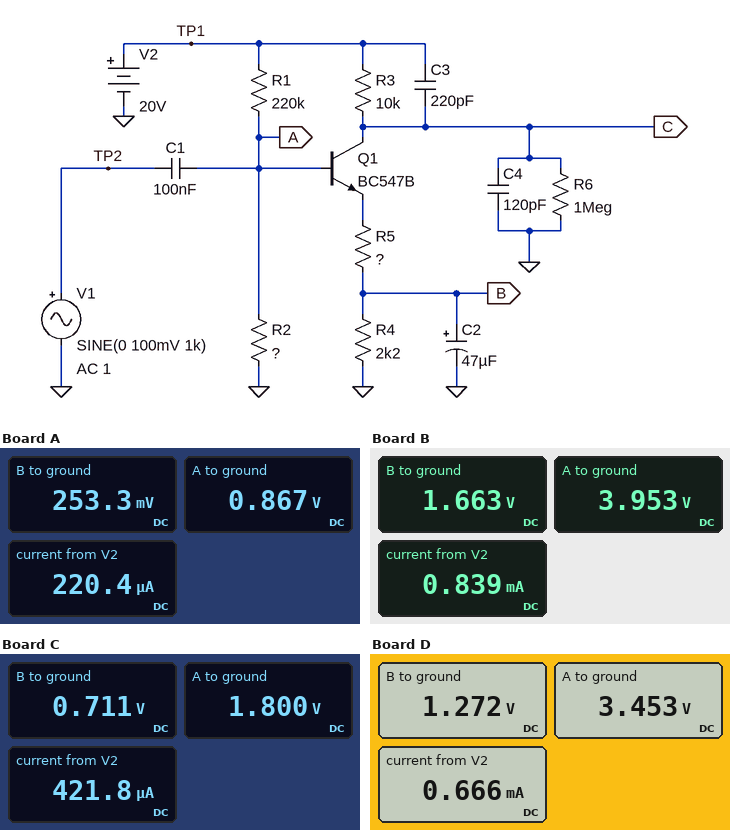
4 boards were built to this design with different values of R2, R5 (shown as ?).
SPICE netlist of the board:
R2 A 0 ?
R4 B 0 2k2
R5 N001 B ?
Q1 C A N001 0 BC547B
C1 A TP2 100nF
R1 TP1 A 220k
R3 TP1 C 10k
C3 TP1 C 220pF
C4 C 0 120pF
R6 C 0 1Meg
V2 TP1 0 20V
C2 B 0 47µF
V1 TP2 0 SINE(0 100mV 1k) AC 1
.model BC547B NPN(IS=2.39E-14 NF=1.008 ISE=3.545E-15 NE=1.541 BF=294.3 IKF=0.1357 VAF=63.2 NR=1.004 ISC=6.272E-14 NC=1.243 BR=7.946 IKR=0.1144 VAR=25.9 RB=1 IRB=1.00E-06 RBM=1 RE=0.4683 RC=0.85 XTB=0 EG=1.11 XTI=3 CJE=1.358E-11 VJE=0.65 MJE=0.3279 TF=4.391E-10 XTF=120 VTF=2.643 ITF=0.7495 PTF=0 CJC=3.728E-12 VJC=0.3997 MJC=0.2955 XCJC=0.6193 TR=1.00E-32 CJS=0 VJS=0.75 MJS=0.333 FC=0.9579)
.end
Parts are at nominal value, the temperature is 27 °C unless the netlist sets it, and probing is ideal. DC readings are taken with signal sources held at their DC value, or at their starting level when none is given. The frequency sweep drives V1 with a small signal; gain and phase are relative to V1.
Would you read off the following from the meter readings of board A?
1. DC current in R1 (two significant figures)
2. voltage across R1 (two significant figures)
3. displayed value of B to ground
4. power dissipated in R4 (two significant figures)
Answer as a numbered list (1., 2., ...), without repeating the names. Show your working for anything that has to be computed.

1. (20 V - 867 mV) / 220 kΩ = 87 µA
2. 20 V - 867 mV = 19 V
3. 253.3 mV
4. (253.3 mV)^2 / 2.2 kΩ = 29 µW
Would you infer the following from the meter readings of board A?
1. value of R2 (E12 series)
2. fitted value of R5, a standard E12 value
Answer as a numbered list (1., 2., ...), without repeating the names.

1. 10 kΩ
2. 330 Ω
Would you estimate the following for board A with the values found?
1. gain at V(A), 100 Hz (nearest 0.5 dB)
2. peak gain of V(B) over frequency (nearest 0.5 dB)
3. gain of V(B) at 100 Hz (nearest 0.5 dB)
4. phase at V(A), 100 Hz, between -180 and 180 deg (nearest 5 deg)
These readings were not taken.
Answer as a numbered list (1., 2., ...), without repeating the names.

1. -6.0 dB
2. -29.5 dB
3. -30.5 dB
4. 60 deg
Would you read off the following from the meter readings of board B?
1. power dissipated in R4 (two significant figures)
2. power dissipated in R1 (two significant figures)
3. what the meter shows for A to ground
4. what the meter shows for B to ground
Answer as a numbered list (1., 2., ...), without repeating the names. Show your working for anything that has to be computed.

1. (1.663 V)^2 / 2.2 kΩ = 1.3 mW
2. (20 V - 3.953 V)^2 / 220 kΩ = 1.2 mW
3. 3.953 V
4. 1.663 V
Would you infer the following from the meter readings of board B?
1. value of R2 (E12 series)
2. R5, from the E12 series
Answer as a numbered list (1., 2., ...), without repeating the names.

1. 56 kΩ
2. 2.2 kΩ
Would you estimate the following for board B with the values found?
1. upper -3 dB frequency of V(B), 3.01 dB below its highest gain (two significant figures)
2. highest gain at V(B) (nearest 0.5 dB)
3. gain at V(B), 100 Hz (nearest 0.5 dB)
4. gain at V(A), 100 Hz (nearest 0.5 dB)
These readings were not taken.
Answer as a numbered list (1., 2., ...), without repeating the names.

1. 44 Hz
2. -28.5 dB
3. -37.0 dB
4. -0.5 dB
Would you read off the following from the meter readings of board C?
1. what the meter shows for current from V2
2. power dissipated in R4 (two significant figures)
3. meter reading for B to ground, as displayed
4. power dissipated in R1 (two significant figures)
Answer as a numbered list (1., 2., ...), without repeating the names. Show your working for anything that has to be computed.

1. 421.8 µA
2. (711 mV)^2 / 2.2 kΩ = 230 µW
3. 0.711 V
4. (20 V - 1.8 V)^2 / 220 kΩ = 1.5 mW
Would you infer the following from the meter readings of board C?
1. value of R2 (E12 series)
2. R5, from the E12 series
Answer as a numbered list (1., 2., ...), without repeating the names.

1. 22 kΩ
2. 1.5 kΩ
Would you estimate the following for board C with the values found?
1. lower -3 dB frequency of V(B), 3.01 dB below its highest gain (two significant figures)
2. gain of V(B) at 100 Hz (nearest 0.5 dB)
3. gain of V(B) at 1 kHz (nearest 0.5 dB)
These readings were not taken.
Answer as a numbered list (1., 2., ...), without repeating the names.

1. 3.3 Hz
2. -35.5 dB
3. -53.5 dB
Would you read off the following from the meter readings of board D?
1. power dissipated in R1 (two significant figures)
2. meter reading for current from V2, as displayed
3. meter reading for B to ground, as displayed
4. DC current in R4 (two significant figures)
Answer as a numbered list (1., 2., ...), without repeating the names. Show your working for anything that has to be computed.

1. (20 V - 3.453 V)^2 / 220 kΩ = 1.2 mW
2. 0.666 mA
3. 1.272 V
4. (1.272 V) / 2.2 kΩ = 580 µA
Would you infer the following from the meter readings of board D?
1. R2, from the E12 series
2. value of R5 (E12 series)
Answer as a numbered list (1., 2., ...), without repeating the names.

1. 47 kΩ
2. 2.7 kΩ
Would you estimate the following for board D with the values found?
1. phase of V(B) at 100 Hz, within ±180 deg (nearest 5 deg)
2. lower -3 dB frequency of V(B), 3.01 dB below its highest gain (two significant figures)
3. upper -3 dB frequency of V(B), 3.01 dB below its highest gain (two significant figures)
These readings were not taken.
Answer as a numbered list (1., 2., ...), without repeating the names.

1. -65 deg
2. 2.4 Hz
3. 48 Hz
